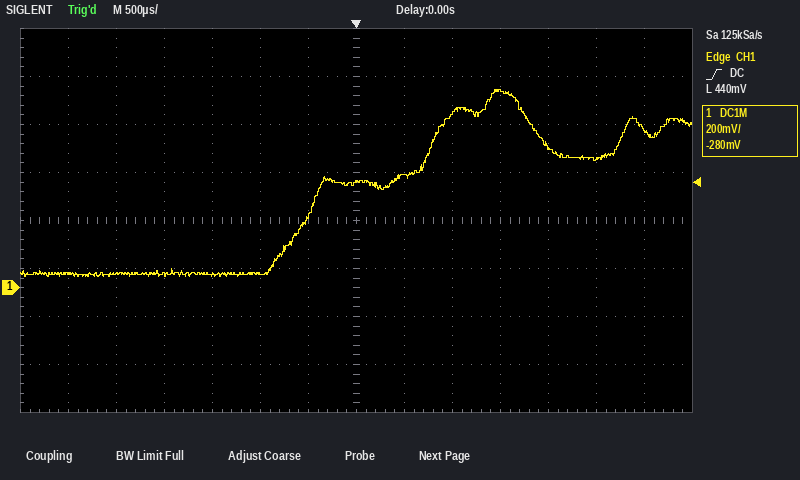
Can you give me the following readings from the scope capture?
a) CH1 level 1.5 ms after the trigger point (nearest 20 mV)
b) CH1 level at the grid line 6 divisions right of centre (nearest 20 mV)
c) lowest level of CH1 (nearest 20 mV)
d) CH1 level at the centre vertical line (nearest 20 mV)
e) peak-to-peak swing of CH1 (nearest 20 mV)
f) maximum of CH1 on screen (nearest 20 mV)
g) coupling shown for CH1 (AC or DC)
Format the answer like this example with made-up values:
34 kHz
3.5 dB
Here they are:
820 mV
660 mV
40 mV
440 mV
780 mV
820 mV
DC
